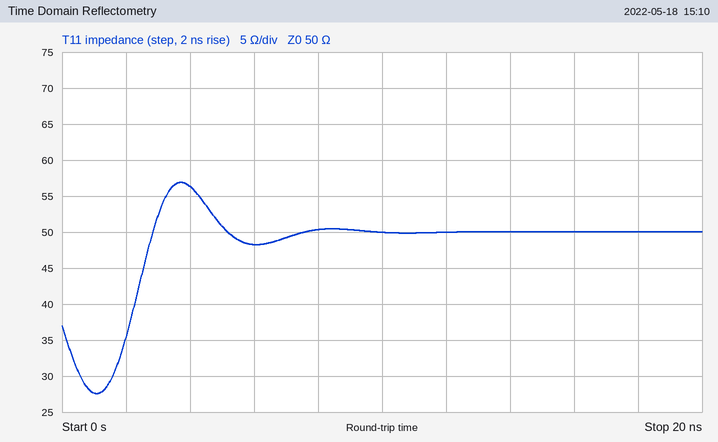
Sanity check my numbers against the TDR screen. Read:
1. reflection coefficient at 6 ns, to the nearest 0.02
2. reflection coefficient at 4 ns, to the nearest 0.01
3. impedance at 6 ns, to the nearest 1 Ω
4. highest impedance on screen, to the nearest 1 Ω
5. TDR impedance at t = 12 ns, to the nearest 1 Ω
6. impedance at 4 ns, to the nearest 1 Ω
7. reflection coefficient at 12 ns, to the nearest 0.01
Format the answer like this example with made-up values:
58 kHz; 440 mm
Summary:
-0.02; +0.06; 48 Ω; 57 Ω; 50 Ω; 56 Ω; 0.00
